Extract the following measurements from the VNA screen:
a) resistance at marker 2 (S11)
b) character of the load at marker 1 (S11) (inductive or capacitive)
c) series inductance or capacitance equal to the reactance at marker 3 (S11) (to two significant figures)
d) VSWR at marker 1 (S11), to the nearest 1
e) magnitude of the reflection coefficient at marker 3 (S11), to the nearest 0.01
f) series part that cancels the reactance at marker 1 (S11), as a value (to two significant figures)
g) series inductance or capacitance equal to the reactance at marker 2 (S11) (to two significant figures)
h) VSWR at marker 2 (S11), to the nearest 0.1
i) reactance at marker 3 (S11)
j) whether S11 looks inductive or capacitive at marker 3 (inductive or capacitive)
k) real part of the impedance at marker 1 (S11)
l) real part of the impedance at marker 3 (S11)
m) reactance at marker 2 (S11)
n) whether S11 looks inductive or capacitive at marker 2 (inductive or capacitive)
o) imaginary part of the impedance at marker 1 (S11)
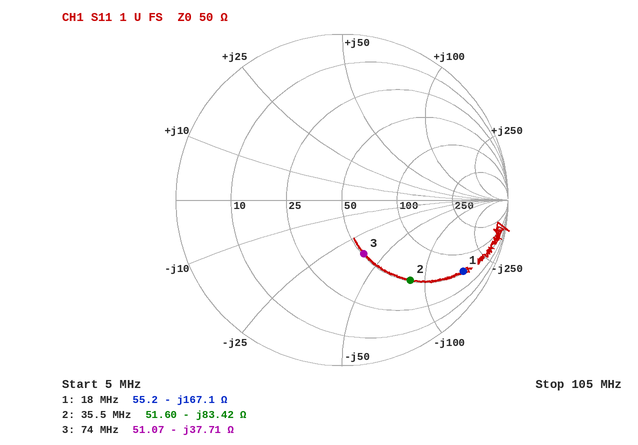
51.60 Ω
capacitive
57 pF
12
0.35
1.5 µH
54 pF
4.5
-37.71 Ω
capacitive
55.2 Ω
51.07 Ω
-83.42 Ω
capacitive
-167.1 Ω
